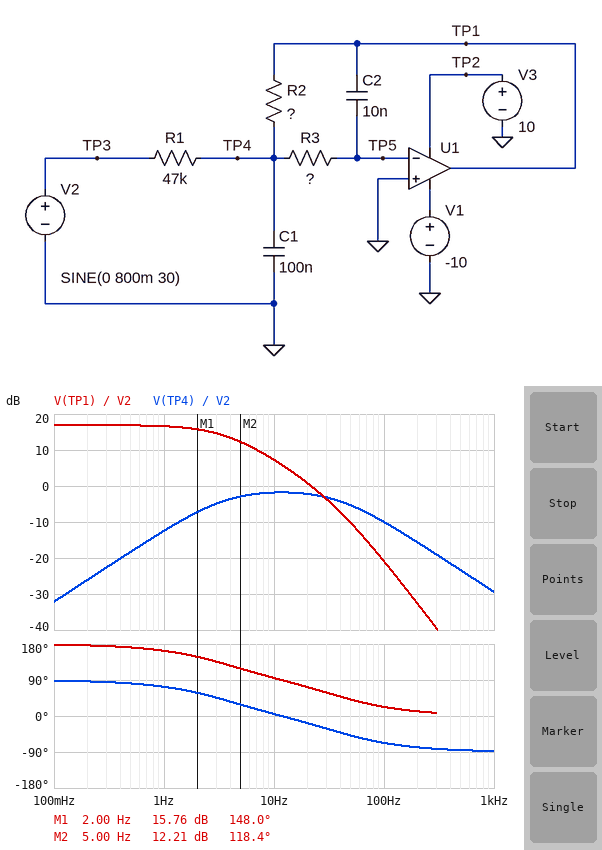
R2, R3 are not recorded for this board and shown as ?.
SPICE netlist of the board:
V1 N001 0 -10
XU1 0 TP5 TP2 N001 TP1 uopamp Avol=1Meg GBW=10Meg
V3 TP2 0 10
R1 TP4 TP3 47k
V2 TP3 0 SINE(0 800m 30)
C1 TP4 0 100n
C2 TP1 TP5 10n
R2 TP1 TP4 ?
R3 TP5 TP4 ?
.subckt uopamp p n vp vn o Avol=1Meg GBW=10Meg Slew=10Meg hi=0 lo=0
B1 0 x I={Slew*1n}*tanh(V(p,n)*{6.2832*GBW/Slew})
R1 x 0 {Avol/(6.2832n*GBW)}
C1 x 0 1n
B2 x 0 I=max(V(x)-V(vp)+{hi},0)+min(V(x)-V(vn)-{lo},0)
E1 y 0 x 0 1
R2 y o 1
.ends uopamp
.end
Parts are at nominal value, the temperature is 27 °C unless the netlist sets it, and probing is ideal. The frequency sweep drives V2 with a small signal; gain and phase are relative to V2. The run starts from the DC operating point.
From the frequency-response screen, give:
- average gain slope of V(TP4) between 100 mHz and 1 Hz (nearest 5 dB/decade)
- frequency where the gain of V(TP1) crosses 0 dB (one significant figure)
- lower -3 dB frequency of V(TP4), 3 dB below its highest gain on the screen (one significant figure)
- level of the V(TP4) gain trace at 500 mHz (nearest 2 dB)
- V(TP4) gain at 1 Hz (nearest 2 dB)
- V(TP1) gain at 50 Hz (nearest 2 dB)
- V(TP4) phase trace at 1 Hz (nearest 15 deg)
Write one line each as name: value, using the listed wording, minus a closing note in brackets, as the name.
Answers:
average gain slope of V(TP4) between 100 mHz and 1 Hz: 20 dB/decade
frequency where the gain of V(TP1) crosses 0 dB: 20 Hz
lower -3 dB frequency of V(TP4), 3 dB below its highest gain on the screen: 3 Hz
level of the V(TP4) gain trace at 500 mHz: -18 dB
V(TP4) gain at 1 Hz: -12 dB
V(TP1) gain at 50 Hz: -10 dB
V(TP4) phase trace at 1 Hz: 75 deg
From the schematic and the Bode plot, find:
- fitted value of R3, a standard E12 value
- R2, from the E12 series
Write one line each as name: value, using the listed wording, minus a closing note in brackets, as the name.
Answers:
fitted value of R3, a standard E12 value: 560 kΩ
R2, from the E12 series: 330 kΩ
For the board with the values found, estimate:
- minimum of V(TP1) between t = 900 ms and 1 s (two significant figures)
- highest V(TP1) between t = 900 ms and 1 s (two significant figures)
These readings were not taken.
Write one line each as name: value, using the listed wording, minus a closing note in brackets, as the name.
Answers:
minimum of V(TP1) between t = 900 ms and 1 s: -530 mV
highest V(TP1) between t = 900 ms and 1 s: 530 mV
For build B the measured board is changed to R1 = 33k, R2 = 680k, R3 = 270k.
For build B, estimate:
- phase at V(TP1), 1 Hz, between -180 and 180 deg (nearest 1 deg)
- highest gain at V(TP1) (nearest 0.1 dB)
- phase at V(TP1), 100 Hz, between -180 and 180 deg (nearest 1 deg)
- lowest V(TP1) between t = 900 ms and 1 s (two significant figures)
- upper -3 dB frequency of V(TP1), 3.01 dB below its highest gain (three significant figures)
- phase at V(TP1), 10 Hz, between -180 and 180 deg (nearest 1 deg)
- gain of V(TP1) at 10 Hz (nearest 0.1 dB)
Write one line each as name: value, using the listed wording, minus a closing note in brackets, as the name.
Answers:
phase at V(TP1), 1 Hz, between -180 and 180 deg: 158 deg
highest gain at V(TP1): 26.3 dB
phase at V(TP1), 100 Hz, between -180 and 180 deg: 30 deg
lowest V(TP1) between t = 900 ms and 1 s: -1.2 V
upper -3 dB frequency of V(TP1), 3.01 dB below its highest gain: 2.55 Hz
phase at V(TP1), 10 Hz, between -180 and 180 deg: 94 deg
gain of V(TP1) at 10 Hz: 14.0 dB
